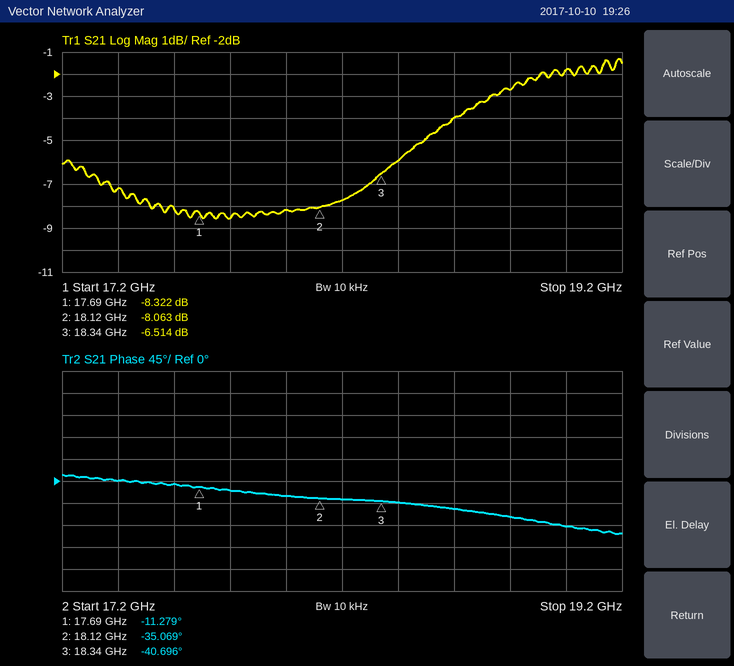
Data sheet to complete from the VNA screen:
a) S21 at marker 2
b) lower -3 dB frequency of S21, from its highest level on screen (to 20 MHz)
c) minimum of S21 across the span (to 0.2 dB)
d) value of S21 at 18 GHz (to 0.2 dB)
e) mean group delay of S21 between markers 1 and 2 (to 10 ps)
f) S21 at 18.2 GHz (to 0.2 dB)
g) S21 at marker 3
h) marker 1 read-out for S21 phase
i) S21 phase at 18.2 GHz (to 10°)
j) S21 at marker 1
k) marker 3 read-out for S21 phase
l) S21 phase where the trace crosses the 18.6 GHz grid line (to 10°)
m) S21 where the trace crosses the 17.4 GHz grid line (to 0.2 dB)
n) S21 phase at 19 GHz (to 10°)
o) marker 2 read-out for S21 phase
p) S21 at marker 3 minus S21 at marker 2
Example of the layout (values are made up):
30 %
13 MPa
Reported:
-8.063 dB
18.56 GHz
-8.6 dB
-8.2 dB
150 ps
-7.8 dB
-6.514 dB
-11.279°
-40°
-8.322 dB
-40.696°
-60°
-7.2 dB
-90°
-35.069°
1.549 dB
